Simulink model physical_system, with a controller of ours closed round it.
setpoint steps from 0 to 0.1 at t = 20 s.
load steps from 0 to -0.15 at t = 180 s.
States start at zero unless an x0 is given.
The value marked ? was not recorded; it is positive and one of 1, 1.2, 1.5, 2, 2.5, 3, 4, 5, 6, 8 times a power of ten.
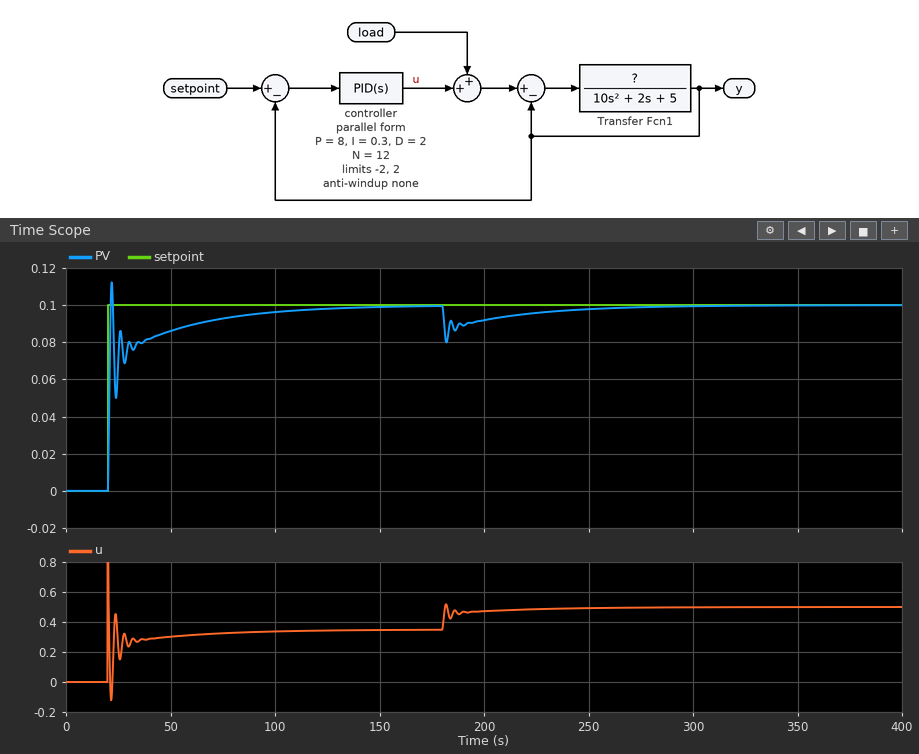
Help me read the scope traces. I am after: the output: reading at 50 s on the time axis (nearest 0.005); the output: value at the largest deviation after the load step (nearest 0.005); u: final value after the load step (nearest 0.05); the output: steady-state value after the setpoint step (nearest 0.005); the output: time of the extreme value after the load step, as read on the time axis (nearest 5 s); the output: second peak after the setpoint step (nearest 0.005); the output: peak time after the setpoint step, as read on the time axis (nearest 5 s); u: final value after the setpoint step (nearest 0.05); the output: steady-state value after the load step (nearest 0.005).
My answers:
0.085
0.080
0.50
0.100
180 s
0.085
20 s
0.35
0.100
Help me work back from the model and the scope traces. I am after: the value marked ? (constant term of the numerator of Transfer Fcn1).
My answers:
2
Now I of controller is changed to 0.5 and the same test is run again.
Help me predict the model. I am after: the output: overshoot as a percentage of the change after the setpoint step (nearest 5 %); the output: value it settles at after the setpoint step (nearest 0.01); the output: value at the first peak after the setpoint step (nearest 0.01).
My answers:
15 %
0.10
0.11
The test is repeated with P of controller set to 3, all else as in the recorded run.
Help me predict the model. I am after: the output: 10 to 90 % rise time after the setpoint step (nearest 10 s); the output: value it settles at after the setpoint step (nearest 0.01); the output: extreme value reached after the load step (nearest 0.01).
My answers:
40 s
0.10
0.07
